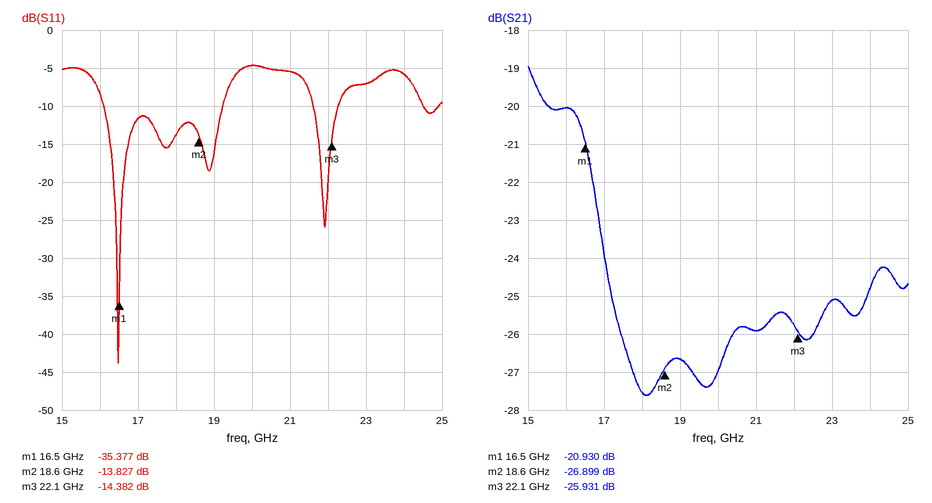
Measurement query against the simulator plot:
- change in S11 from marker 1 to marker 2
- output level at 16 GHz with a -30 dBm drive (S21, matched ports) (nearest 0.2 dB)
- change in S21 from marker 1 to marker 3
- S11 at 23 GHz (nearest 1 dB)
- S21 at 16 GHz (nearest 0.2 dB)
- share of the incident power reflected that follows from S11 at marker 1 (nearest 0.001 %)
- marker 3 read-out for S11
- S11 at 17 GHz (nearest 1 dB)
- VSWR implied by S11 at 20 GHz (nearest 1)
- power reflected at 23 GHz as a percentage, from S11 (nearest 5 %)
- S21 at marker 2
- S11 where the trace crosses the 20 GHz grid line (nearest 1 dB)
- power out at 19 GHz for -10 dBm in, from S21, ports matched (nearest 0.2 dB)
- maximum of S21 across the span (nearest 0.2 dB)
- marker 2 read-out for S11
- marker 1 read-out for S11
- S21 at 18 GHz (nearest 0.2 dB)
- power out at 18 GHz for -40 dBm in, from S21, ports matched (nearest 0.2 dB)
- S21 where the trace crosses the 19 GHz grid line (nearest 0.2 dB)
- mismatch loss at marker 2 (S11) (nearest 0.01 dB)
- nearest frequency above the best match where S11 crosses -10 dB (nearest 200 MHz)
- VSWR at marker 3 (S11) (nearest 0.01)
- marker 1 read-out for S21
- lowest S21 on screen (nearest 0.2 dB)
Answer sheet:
21.550 dB
-50.0 dBm
-5.001 dB
-7 dB
-20.0 dB
0.029 %
-14.382 dB
-12 dB
4
20 %
-26.899 dB
-5 dB
-36.6 dBm
-19.0 dB
-13.827 dB
-35.377 dB
-27.6 dB
-67.6 dBm
-26.6 dB
0.18 dB
19.2 GHz
1.47
-20.930 dB
-27.6 dB
